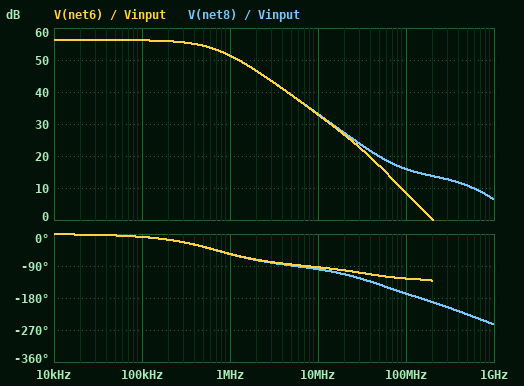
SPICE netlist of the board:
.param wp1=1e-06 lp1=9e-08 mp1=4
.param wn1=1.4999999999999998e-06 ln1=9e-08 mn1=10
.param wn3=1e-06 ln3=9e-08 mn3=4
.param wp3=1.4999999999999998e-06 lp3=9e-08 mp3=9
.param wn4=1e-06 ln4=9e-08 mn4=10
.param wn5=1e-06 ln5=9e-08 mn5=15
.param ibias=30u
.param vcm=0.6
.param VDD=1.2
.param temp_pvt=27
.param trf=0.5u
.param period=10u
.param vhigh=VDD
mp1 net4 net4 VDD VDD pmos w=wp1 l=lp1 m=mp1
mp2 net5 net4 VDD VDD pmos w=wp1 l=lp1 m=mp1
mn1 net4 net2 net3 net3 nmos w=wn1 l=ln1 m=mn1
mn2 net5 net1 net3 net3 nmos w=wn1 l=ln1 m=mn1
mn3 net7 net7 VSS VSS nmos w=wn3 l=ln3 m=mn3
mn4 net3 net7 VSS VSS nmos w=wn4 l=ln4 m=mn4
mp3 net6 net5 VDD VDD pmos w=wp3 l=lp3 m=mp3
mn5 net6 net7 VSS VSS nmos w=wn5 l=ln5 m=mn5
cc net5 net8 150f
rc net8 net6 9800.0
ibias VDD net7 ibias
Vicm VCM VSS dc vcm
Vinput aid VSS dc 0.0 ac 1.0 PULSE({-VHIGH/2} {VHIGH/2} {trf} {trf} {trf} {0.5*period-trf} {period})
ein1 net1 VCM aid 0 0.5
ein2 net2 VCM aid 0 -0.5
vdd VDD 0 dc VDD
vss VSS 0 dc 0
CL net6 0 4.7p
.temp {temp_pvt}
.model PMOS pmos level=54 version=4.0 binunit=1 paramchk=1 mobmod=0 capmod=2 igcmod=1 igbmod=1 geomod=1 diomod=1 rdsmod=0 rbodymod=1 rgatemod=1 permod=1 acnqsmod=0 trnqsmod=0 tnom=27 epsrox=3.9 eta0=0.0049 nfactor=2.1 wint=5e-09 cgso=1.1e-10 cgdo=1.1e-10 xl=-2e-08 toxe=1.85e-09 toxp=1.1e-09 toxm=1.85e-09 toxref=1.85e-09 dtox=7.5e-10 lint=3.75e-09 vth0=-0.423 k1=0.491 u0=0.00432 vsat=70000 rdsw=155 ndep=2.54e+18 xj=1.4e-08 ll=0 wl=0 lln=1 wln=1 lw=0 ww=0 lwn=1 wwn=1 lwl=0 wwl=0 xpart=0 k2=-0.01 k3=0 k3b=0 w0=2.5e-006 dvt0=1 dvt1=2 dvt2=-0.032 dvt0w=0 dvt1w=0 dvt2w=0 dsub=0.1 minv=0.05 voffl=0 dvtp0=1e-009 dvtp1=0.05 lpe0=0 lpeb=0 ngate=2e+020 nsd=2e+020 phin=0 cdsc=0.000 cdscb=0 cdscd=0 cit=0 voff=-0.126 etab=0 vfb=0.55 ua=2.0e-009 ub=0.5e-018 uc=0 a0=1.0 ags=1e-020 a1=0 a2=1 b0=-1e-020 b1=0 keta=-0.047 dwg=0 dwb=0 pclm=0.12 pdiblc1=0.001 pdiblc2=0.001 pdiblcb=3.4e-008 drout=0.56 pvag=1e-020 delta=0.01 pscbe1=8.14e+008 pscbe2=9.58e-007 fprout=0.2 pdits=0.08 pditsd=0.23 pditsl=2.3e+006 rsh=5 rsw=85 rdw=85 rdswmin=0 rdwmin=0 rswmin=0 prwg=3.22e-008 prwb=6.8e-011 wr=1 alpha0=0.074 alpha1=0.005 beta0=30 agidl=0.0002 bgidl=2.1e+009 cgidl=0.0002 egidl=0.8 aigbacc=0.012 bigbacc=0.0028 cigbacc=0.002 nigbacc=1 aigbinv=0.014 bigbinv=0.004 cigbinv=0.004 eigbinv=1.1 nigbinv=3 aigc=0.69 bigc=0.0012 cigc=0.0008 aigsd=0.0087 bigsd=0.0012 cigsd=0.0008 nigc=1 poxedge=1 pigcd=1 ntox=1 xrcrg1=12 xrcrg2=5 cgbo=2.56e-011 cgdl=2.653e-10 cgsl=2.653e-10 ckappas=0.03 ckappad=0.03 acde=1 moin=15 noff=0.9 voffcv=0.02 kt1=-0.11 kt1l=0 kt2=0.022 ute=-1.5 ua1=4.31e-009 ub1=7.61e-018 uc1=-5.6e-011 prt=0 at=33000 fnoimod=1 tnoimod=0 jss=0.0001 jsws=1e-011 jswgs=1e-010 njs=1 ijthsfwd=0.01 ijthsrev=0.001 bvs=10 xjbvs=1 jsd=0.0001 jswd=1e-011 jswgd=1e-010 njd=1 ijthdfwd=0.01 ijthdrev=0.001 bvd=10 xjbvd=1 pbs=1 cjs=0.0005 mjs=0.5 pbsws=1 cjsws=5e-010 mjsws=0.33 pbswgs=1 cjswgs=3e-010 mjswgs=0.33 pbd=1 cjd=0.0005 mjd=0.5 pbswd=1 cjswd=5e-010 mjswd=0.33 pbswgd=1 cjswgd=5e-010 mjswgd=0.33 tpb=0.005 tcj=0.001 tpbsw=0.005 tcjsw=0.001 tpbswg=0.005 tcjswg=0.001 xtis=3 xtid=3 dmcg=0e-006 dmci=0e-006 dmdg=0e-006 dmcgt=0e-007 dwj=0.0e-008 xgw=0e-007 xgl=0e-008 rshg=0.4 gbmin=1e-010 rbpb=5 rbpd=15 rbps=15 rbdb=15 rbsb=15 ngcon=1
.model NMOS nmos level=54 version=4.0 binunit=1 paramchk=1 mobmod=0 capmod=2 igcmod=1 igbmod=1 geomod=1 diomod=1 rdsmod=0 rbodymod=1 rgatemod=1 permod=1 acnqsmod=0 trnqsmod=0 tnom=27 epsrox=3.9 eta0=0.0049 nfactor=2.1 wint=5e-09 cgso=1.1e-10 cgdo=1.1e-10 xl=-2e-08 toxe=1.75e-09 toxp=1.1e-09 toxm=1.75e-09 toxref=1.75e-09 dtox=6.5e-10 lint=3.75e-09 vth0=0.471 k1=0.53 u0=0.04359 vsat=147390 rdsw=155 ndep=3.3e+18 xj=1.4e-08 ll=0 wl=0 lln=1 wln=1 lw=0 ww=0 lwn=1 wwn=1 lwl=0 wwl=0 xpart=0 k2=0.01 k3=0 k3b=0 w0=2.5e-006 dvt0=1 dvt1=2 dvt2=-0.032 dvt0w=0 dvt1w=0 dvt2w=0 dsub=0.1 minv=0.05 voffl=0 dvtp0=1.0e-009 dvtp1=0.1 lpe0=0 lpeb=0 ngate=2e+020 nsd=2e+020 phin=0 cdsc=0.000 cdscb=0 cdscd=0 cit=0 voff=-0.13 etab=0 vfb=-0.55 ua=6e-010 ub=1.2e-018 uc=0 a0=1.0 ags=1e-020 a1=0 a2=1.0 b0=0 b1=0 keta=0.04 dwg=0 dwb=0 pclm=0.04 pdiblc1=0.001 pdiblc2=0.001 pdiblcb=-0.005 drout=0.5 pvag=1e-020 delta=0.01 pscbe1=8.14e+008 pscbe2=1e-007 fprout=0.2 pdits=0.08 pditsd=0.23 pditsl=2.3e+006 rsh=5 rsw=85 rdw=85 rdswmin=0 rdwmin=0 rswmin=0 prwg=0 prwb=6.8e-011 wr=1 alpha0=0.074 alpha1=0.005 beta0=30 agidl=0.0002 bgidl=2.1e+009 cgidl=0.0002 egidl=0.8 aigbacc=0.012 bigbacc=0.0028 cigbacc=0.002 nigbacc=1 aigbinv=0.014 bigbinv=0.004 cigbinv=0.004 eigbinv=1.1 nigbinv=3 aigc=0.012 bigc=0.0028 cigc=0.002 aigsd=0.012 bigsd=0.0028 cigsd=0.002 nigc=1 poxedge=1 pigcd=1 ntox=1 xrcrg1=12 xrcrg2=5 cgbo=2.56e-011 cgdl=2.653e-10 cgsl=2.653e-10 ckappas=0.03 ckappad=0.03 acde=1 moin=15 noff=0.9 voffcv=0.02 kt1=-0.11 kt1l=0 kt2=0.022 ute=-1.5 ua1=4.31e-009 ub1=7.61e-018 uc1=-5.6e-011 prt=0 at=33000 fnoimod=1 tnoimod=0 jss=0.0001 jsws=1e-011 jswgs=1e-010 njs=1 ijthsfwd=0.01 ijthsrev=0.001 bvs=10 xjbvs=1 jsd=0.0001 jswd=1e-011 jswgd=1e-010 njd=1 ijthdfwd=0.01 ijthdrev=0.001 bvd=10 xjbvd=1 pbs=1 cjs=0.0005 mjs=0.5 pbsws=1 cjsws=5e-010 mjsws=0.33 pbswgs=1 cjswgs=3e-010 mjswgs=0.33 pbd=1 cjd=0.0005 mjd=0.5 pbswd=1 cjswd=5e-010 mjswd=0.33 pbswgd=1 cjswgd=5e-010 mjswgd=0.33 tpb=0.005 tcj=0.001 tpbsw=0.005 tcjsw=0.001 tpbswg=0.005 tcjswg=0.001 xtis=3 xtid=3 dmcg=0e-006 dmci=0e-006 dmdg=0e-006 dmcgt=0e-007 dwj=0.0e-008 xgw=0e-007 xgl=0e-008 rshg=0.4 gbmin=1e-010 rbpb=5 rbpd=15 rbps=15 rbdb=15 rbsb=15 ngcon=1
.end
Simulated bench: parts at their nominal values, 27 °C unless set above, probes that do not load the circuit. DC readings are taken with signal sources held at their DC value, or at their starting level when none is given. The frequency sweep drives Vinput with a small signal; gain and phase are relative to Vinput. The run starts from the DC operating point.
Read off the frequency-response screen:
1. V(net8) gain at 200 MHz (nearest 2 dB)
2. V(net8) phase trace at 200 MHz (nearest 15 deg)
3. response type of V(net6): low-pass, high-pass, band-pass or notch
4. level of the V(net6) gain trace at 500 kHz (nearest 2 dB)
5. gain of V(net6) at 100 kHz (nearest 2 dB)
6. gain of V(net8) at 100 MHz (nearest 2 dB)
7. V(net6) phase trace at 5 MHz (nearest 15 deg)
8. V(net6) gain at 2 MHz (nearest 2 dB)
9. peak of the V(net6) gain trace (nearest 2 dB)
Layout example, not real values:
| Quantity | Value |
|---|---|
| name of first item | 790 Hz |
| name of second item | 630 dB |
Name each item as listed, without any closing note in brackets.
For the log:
| Quantity | Value |
|---|---|
| V(net8) gain at 200 MHz | 14 dB |
| V(net8) phase trace at 200 MHz | -195 deg |
| response type of V(net6): low-pass, high-pass, band-pass or notch | low-pass |
| level of the V(net6) gain trace at 500 kHz | 54 dB |
| gain of V(net6) at 100 kHz | 56 dB |
| gain of V(net8) at 100 MHz | 16 dB |
| V(net6) phase trace at 5 MHz | -90 deg |
| V(net6) gain at 2 MHz | 46 dB |
| peak of the V(net6) gain trace | 56 dB |
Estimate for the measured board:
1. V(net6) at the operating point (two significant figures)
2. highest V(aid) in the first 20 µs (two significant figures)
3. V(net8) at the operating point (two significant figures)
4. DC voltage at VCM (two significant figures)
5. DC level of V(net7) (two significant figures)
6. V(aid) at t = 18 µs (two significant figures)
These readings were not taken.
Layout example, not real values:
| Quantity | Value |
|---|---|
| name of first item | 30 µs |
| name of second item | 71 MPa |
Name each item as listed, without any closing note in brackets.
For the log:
| Quantity | Value |
|---|---|
| V(net6) at the operating point | 620 mV |
| highest V(aid) in the first 20 µs | 600 mV |
| V(net8) at the operating point | 620 mV |
| DC voltage at VCM | 600 mV |
| DC level of V(net7) | 430 mV |
| V(aid) at t = 18 µs | -600 mV |
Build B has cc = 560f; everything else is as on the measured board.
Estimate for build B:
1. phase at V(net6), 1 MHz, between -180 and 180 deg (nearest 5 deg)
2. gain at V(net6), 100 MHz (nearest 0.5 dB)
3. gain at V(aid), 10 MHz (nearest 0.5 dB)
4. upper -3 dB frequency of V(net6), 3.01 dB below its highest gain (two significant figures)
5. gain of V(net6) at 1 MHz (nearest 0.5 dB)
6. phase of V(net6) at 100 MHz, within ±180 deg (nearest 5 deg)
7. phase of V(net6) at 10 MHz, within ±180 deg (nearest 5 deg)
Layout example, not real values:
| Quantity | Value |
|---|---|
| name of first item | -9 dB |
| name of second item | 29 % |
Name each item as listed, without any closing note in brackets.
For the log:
| Quantity | Value |
|---|---|
| phase at V(net6), 1 MHz, between -180 and 180 deg | -75 deg |
| gain at V(net6), 100 MHz | 6.5 dB |
| gain at V(aid), 10 MHz | 0 dB |
| upper -3 dB frequency of V(net6), 3.01 dB below its highest gain | 250 kHz |
| gain of V(net6) at 1 MHz | 44.0 dB |
| phase of V(net6) at 100 MHz, within ±180 deg | -100 deg |
| phase of V(net6) at 10 MHz, within ±180 deg | -85 deg |
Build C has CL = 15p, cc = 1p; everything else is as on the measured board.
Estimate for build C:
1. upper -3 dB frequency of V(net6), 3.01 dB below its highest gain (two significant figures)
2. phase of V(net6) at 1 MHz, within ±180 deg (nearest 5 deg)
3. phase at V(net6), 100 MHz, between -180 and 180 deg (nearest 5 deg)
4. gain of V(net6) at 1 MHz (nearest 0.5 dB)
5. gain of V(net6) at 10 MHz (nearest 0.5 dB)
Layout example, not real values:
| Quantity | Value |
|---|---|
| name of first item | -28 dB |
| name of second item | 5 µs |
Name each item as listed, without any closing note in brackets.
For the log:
| Quantity | Value |
|---|---|
| upper -3 dB frequency of V(net6), 3.01 dB below its highest gain | 130 kHz |
| phase of V(net6) at 1 MHz, within ±180 deg | -85 deg |
| phase at V(net6), 100 MHz, between -180 and 180 deg | -105 deg |
| gain of V(net6) at 1 MHz | 38.5 dB |
| gain of V(net6) at 10 MHz | 18.0 dB |
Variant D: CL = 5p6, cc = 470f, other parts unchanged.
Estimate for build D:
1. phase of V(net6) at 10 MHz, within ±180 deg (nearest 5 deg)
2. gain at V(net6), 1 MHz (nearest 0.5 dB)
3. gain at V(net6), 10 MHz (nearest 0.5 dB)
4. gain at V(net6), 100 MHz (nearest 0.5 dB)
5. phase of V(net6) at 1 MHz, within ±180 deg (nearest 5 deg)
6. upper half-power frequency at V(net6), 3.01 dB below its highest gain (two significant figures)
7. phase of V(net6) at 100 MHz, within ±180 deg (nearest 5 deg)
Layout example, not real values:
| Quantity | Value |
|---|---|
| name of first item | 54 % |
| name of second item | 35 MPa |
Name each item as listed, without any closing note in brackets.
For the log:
| Quantity | Value |
|---|---|
| phase of V(net6) at 10 MHz, within ±180 deg | -90 deg |
| gain at V(net6), 1 MHz | 45.0 dB |
| gain at V(net6), 10 MHz | 25.0 dB |
| gain at V(net6), 100 MHz | 5.0 dB |
| phase of V(net6) at 1 MHz, within ±180 deg | -75 deg |
| upper half-power frequency at V(net6), 3.01 dB below its highest gain | 280 kHz |
| phase of V(net6) at 100 MHz, within ±180 deg | -105 deg |
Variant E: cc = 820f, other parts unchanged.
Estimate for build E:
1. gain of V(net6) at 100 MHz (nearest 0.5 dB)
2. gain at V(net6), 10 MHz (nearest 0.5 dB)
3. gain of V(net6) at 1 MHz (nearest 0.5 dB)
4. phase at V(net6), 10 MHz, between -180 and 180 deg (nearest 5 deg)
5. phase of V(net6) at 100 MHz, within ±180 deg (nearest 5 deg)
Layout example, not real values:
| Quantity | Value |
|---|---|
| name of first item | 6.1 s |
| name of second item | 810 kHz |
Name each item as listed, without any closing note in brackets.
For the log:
| Quantity | Value |
|---|---|
| gain of V(net6) at 100 MHz | 6.5 dB |
| gain at V(net6), 10 MHz | 21.5 dB |
| gain of V(net6) at 1 MHz | 41.0 dB |
| phase at V(net6), 10 MHz, between -180 and 180 deg | -80 deg |
| phase of V(net6) at 100 MHz, within ±180 deg | -95 deg |
